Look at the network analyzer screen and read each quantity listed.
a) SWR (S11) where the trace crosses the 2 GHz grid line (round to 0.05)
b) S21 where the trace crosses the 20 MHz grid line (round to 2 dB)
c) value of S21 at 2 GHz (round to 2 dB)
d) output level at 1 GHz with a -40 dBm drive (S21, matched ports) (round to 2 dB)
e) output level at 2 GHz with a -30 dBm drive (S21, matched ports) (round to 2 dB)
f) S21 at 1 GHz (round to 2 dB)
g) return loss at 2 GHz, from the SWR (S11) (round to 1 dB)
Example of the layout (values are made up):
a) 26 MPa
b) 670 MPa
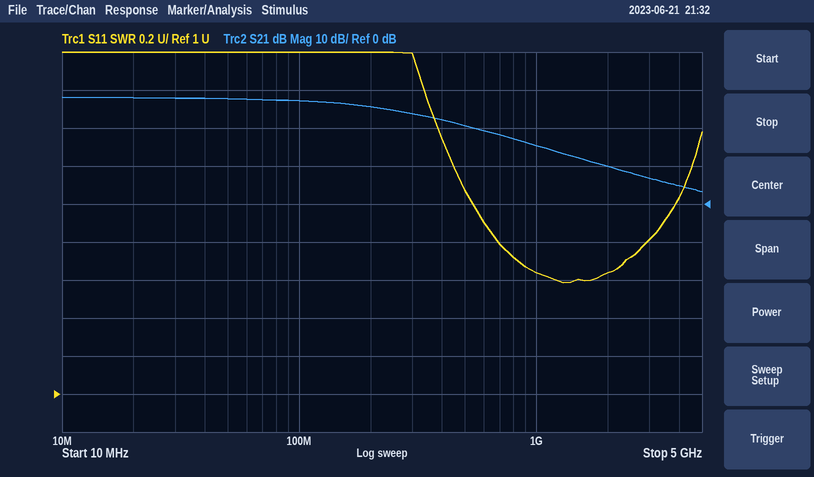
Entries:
a) 1.65
b) 28 dB
c) 10 dB
d) -24 dBm
e) -20 dBm
f) 16 dB
g) 12 dB
